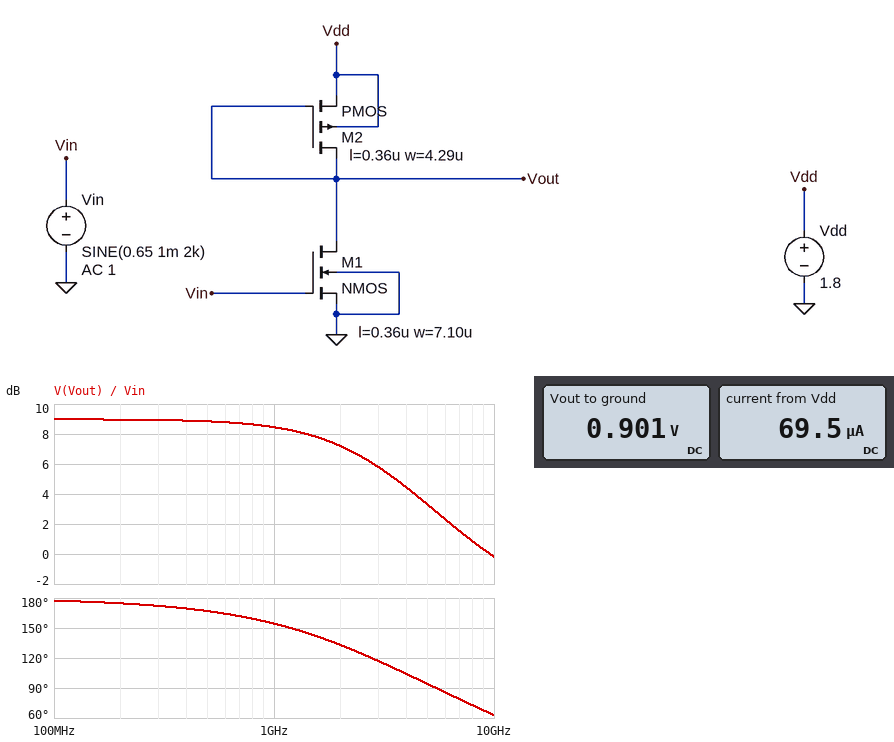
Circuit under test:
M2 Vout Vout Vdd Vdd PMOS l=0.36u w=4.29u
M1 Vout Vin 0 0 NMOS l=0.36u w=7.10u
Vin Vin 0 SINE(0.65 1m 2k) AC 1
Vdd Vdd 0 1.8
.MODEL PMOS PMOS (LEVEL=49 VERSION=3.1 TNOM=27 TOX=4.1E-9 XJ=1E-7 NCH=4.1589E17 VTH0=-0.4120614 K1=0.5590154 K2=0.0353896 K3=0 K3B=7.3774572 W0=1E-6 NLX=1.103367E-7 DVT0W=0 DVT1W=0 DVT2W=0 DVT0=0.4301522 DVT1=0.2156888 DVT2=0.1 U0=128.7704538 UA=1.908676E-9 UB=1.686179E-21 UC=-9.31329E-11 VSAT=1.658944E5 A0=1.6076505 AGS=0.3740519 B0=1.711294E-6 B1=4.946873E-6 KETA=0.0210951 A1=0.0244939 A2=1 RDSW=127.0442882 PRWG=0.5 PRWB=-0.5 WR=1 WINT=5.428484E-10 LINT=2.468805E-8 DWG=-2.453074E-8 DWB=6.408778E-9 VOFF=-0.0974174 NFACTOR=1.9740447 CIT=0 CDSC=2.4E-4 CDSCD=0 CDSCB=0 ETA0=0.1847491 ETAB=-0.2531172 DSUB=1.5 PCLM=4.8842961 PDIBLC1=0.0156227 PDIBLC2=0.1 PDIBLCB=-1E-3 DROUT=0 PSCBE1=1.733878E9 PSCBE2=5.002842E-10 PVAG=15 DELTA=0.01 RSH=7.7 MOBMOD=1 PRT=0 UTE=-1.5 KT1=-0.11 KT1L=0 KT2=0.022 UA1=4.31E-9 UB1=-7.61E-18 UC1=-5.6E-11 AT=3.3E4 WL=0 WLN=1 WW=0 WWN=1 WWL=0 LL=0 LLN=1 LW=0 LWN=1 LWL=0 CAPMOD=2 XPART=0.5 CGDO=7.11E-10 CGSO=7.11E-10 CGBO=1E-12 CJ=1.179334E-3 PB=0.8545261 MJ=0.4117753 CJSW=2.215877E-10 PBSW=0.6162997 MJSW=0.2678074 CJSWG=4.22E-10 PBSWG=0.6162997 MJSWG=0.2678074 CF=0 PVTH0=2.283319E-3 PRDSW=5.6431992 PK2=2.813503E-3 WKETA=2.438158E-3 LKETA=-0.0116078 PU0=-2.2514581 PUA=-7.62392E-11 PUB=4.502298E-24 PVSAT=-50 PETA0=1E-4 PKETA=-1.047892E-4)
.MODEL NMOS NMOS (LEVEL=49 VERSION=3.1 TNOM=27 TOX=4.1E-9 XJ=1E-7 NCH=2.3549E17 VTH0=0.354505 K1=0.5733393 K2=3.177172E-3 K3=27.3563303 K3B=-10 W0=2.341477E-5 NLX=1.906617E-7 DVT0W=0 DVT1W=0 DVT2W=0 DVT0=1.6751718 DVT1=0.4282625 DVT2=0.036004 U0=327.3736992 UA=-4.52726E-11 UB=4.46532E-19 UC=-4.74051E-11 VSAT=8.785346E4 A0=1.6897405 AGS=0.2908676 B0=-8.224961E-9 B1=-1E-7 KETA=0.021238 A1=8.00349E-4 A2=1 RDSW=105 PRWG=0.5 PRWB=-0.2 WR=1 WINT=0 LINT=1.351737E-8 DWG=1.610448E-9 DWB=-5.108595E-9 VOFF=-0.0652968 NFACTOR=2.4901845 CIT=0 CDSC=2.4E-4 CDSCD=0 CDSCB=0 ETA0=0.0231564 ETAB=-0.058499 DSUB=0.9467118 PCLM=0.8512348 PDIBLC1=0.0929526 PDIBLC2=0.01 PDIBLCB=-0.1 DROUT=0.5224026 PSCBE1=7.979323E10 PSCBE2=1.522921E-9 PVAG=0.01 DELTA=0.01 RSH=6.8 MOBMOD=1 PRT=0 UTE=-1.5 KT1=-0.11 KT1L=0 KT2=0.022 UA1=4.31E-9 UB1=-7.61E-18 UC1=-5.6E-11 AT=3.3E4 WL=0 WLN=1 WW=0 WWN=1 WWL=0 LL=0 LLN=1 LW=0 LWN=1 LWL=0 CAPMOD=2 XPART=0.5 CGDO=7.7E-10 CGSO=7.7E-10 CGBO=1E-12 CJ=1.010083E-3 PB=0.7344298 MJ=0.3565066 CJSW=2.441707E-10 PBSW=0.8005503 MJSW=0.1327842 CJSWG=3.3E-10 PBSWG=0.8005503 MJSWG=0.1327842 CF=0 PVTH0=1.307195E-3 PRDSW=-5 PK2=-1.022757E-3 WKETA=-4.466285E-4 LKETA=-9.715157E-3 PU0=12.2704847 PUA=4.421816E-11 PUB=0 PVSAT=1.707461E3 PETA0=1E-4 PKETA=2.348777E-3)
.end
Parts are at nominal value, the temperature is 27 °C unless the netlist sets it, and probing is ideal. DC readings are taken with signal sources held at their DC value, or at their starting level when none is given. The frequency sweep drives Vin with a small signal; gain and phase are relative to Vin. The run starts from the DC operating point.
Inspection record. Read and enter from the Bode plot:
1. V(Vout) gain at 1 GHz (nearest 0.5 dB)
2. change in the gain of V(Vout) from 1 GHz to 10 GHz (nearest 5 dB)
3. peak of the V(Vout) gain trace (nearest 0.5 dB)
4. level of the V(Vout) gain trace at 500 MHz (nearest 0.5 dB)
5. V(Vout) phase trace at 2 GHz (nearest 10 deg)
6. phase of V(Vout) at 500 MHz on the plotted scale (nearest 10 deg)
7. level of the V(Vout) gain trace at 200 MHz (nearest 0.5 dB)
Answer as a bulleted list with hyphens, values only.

- 8.5 dB
- -10 dB
- 9.0 dB
- 9.0 dB
- 130 deg
- 170 deg
- 9.0 dB
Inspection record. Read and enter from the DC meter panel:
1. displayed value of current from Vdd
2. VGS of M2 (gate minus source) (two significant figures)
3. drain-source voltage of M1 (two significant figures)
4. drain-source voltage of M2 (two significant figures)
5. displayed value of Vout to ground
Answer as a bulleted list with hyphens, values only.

- 69.5 µA
- -900 mV
- 900 mV
- -900 mV
- 0.901 V
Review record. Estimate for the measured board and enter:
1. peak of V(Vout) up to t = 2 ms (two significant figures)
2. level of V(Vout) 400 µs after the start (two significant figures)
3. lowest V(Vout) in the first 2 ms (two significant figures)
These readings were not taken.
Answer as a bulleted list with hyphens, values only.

- 900 mV
- 900 mV
- 900 mV
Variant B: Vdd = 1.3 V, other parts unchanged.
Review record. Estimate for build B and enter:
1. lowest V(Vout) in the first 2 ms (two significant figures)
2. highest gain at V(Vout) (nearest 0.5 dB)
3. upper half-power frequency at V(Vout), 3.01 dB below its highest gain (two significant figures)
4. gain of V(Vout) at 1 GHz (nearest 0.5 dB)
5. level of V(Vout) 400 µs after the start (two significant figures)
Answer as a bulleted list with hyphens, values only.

- 410 mV
- 8.5 dB
- 2.8 GHz
- 8.0 dB
- 420 mV
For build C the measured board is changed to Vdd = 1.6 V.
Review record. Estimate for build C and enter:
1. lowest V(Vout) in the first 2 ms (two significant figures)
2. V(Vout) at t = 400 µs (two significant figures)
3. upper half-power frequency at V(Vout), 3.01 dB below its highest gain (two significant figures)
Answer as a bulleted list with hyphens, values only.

- 700 mV
- 710 mV
- 2.8 GHz
